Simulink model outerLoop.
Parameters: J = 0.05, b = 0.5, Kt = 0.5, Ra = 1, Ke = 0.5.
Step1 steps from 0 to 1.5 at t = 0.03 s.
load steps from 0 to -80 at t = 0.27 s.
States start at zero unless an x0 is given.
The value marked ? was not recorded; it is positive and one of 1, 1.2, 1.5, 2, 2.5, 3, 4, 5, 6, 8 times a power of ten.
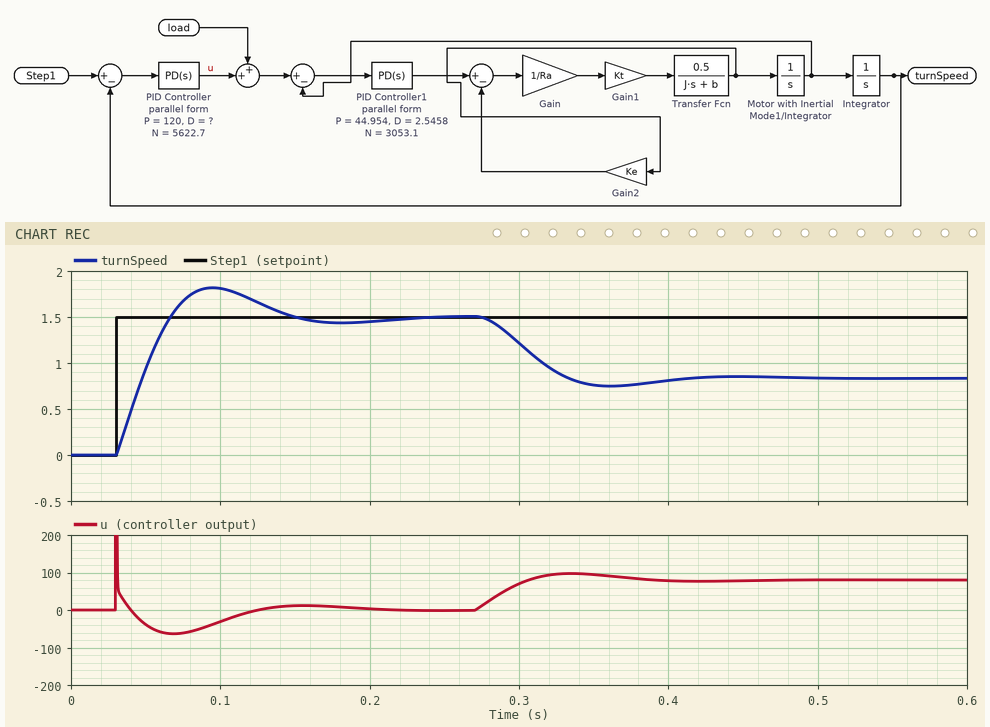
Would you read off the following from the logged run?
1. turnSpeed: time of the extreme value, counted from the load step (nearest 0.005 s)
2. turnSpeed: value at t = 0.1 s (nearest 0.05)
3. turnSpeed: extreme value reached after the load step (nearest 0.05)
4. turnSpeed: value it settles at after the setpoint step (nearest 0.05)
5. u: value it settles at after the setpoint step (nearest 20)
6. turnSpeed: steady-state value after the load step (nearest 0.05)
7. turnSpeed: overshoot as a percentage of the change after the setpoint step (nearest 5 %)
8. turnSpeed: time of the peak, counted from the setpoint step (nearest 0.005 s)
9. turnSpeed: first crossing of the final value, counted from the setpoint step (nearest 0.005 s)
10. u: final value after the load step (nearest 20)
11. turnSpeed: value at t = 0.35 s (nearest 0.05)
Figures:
0.090 s
1.80
0.75
1.50
0
0.85
20 %
0.065 s
0.035 s
80
0.75
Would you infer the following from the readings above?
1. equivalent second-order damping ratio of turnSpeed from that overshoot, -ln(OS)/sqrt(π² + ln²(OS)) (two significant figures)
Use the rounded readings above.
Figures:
0.46
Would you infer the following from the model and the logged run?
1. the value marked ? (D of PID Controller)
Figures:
2.5
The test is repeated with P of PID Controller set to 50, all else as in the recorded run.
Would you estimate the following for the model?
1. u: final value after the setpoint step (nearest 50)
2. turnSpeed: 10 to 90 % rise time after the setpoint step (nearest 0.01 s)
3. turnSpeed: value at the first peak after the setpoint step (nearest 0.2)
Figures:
0
0.04 s
1.6
